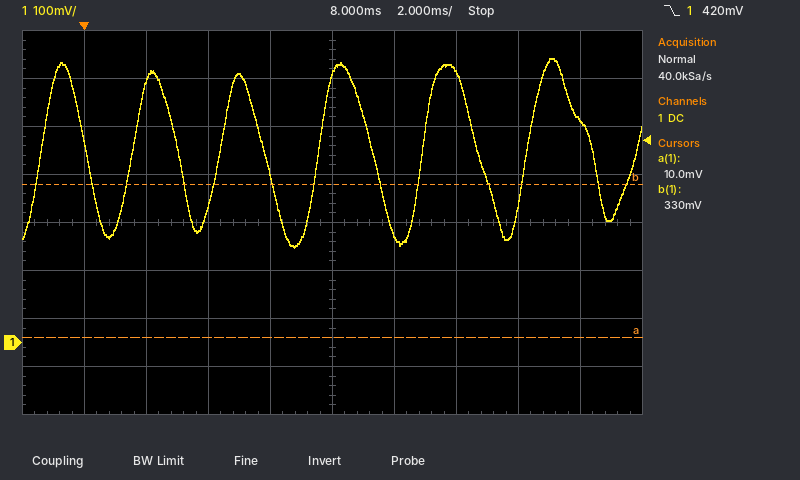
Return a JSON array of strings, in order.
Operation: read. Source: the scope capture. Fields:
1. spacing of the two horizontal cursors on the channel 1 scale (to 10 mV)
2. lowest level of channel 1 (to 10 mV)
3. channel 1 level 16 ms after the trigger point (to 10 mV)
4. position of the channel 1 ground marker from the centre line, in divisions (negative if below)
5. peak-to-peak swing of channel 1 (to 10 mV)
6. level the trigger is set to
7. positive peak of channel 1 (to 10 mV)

["320 mV", "200 mV", "460 mV", "-2.5 div", "390 mV", "420 mV", "590 mV"]
